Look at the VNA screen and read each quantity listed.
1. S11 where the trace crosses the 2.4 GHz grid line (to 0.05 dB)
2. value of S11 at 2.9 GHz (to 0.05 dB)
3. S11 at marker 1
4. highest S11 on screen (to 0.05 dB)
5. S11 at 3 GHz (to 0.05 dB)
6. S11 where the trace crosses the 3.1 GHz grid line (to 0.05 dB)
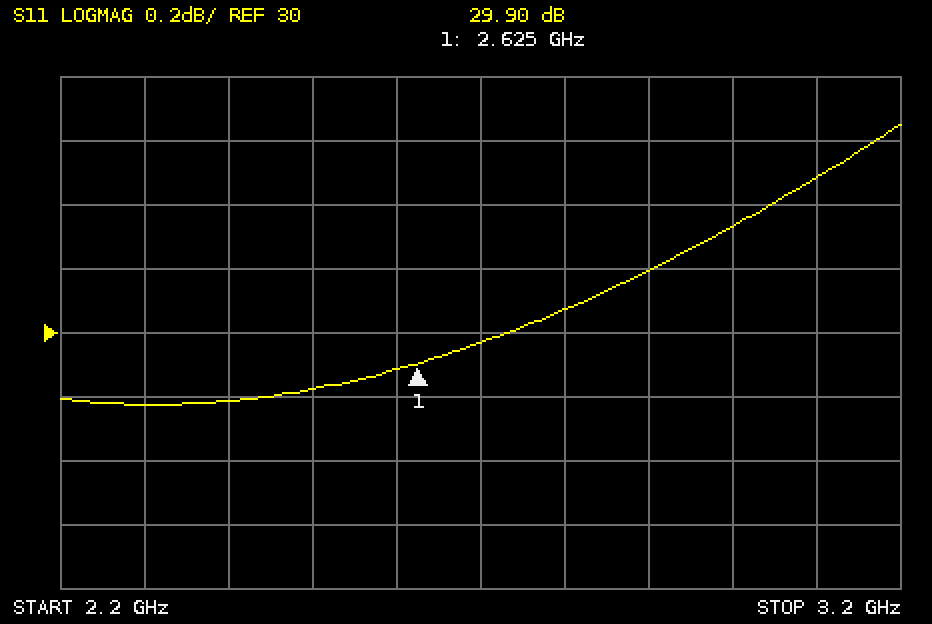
29.80 dB
30.20 dB
29.90 dB
30.65 dB
30.35 dB
30.50 dB
